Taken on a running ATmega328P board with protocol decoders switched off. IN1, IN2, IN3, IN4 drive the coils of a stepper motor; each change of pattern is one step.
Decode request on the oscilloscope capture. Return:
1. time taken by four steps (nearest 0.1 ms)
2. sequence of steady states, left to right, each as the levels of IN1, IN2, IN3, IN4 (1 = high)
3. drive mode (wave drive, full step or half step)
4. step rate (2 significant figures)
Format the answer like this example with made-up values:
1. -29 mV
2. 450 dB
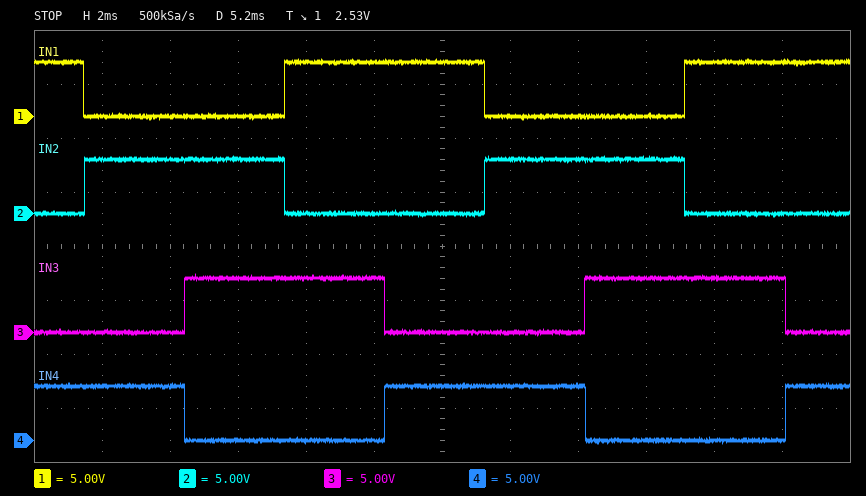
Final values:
1. 11.8 ms
2. 1001 0101 0110 1010 1001 0101 0110 1010 1001
3. full step
4. 340 steps/s
